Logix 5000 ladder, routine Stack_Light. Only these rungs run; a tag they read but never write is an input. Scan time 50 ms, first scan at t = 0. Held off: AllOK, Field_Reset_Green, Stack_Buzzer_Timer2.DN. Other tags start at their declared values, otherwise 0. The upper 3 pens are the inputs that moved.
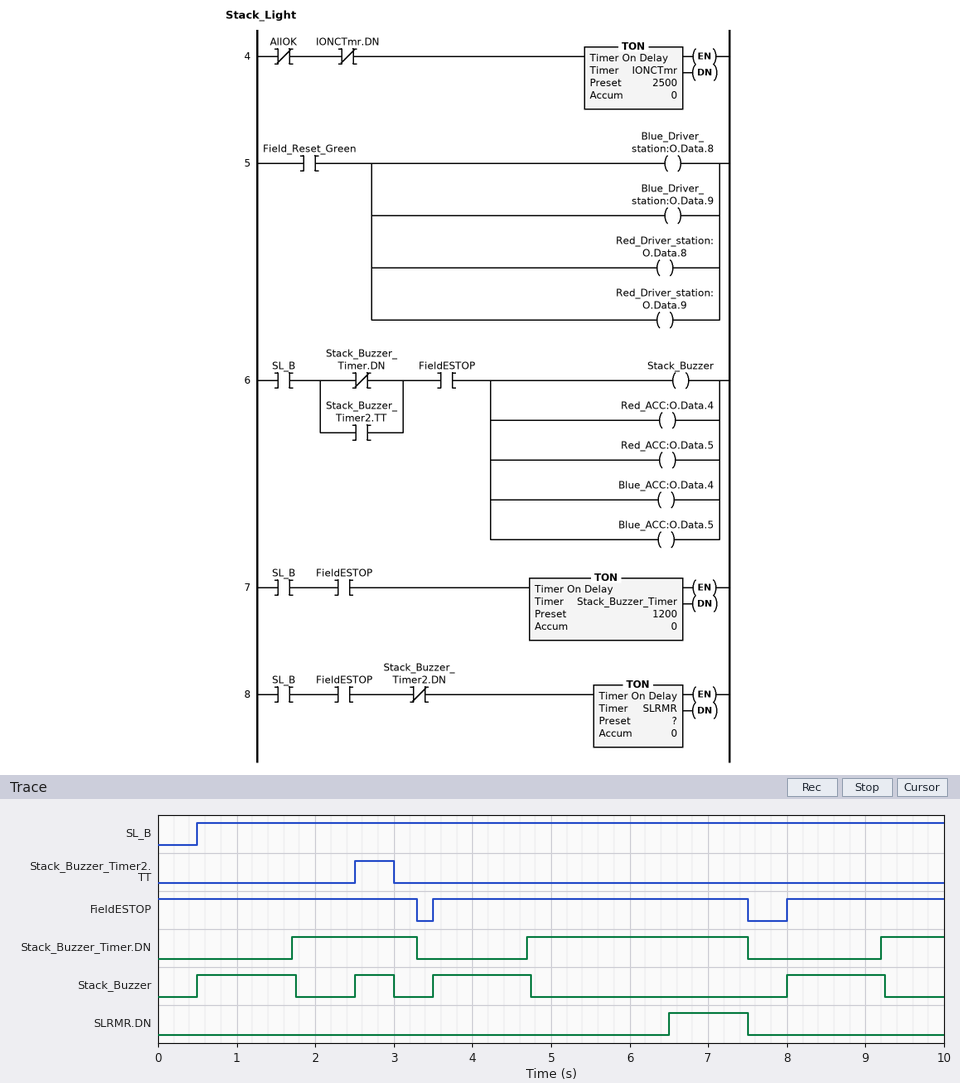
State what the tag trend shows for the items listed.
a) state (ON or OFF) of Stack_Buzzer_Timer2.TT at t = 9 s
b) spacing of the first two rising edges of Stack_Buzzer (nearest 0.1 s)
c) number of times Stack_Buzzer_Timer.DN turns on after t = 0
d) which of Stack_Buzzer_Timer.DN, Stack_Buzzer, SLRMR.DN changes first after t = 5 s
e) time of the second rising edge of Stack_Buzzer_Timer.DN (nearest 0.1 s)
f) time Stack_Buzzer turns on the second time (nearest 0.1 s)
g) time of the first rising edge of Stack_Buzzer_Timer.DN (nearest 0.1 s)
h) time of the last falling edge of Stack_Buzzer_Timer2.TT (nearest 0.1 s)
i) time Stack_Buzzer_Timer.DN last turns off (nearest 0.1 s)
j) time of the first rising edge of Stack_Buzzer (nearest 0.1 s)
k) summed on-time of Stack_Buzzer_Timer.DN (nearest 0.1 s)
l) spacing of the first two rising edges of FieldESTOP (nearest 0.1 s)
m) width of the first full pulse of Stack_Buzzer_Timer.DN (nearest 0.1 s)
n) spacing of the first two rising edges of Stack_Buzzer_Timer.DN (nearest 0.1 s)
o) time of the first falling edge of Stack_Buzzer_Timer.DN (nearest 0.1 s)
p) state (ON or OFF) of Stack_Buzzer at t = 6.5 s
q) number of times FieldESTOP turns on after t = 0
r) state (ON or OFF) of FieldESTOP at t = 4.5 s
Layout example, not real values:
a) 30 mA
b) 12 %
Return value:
a) OFF
b) 2.0 s
c) 3
d) SLRMR.DN
e) 4.7 s
f) 2.5 s
g) 1.7 s
h) 3.0 s
i) 7.5 s
j) 0.5 s
k) 5.2 s
l) 4.5 s
m) 1.6 s
n) 3.0 s
o) 3.3 s
p) OFF
q) 2
r) ON
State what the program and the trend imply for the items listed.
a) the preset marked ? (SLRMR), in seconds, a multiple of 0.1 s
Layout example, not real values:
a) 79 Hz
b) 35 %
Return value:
a) 3.0 s
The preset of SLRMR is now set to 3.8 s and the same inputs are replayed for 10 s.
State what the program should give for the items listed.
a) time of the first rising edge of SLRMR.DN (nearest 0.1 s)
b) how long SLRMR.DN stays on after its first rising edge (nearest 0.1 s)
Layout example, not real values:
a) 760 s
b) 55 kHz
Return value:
a) 7.3 s
b) 0.2 s
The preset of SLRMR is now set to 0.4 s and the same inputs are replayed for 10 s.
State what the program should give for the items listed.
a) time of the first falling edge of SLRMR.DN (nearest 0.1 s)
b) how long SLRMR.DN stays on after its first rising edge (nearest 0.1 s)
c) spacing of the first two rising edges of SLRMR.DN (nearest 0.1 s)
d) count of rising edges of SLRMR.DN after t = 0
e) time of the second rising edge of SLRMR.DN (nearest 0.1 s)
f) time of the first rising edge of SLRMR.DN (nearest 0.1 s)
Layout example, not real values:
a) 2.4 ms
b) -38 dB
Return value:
a) 3.3 s
b) 2.4 s
c) 3.0 s
d) 3
e) 3.9 s
f) 0.9 s
